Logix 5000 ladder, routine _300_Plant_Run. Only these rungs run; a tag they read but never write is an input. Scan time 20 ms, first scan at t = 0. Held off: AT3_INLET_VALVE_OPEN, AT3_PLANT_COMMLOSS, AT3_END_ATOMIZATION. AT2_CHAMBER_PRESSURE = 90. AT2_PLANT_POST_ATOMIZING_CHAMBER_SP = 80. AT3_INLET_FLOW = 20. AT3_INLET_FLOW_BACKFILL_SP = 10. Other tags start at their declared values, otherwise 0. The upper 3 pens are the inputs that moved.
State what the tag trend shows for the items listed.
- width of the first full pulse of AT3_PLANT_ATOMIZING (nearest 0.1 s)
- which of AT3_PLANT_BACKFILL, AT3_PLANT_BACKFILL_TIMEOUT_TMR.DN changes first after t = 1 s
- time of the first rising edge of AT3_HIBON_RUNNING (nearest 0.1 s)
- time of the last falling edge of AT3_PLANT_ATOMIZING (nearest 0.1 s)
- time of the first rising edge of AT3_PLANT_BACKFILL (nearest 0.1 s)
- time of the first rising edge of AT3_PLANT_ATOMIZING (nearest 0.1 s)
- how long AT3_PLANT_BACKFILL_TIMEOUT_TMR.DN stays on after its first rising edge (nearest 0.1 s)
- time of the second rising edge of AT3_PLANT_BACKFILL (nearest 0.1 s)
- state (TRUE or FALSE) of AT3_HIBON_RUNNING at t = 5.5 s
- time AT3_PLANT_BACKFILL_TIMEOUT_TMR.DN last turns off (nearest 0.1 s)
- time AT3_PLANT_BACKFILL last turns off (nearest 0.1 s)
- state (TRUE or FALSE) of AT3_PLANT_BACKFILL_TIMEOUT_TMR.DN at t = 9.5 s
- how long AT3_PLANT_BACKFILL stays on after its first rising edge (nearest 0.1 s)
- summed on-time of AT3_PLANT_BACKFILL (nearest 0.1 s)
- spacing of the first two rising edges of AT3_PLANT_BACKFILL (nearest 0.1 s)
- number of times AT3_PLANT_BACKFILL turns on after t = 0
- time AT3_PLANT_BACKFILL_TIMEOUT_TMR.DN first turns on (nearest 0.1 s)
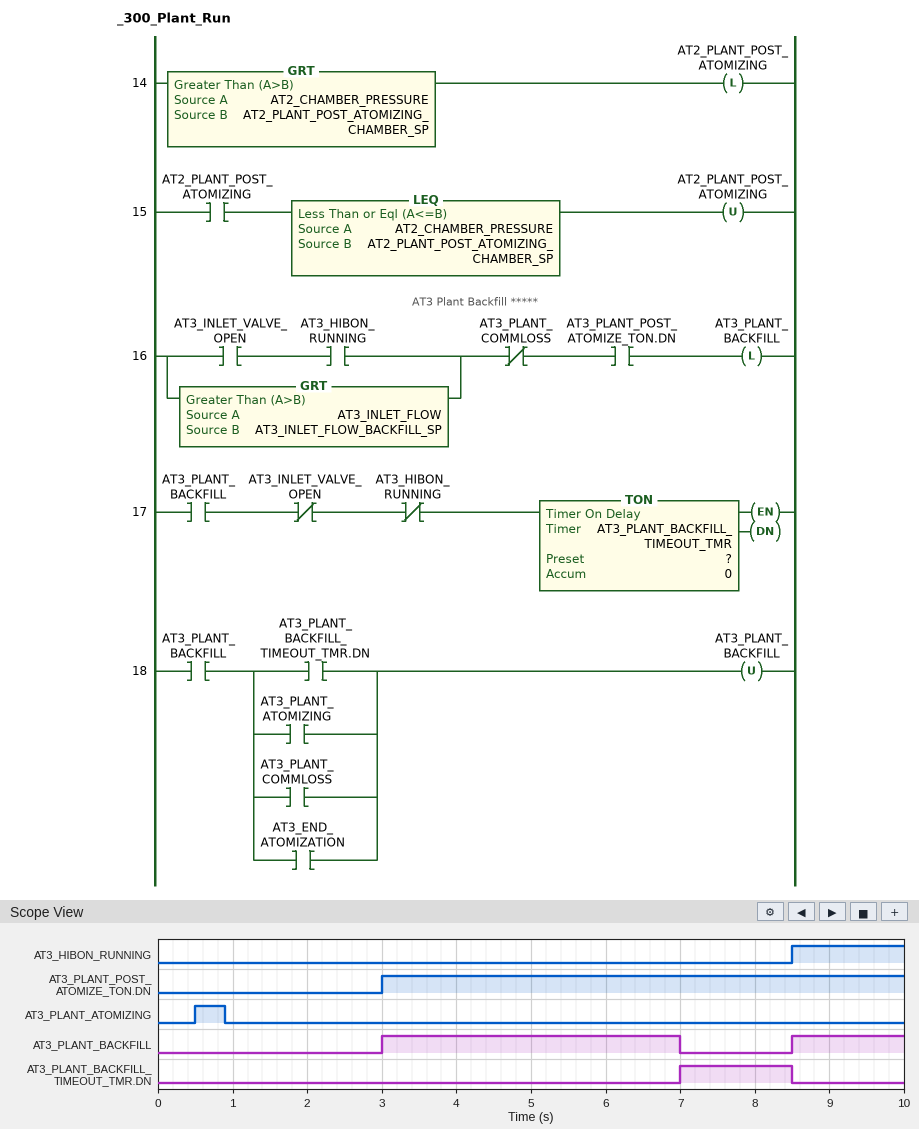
0.4 s
AT3_PLANT_BACKFILL
8.5 s
0.9 s
3.0 s
0.5 s
1.5 s
8.5 s
FALSE
8.5 s
7.0 s
FALSE
4.0 s
5.5 s
5.5 s
2
7.0 s
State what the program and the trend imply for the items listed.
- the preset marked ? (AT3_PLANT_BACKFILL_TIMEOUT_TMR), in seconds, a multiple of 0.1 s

4.0 s
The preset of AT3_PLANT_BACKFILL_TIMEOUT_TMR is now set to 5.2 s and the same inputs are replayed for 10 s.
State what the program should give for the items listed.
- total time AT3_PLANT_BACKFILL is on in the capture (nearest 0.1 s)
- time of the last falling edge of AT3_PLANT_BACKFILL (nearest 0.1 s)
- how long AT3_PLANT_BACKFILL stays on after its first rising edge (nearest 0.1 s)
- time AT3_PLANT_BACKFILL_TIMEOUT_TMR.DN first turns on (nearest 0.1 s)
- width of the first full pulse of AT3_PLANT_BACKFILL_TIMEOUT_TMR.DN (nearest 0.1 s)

6.7 s
8.2 s
5.2 s
8.2 s
0.3 s
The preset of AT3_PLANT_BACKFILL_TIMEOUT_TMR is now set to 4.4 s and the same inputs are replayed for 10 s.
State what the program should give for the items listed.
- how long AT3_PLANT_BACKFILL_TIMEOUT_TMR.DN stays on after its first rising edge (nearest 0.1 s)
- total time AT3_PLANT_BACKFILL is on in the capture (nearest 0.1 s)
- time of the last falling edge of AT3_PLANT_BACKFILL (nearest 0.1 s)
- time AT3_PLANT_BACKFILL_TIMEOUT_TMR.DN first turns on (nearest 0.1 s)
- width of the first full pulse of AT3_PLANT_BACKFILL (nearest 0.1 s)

1.1 s
5.9 s
7.4 s
7.4 s
4.4 s
